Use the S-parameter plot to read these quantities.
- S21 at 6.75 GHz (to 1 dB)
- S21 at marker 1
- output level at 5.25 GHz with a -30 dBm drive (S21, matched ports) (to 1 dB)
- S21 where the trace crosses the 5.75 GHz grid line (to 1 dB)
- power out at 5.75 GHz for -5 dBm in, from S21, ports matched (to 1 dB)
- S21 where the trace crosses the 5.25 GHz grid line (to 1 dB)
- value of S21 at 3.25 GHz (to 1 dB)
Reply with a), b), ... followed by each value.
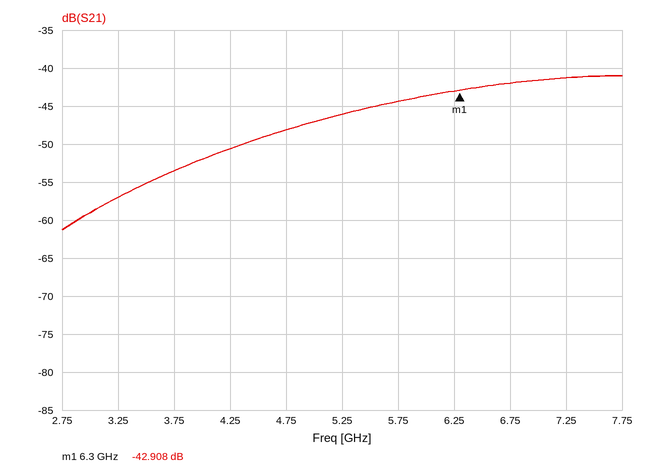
a) -42 dB
b) -42.908 dB
c) -76 dBm
d) -44 dB
e) -49 dBm
f) -46 dB
g) -57 dB
